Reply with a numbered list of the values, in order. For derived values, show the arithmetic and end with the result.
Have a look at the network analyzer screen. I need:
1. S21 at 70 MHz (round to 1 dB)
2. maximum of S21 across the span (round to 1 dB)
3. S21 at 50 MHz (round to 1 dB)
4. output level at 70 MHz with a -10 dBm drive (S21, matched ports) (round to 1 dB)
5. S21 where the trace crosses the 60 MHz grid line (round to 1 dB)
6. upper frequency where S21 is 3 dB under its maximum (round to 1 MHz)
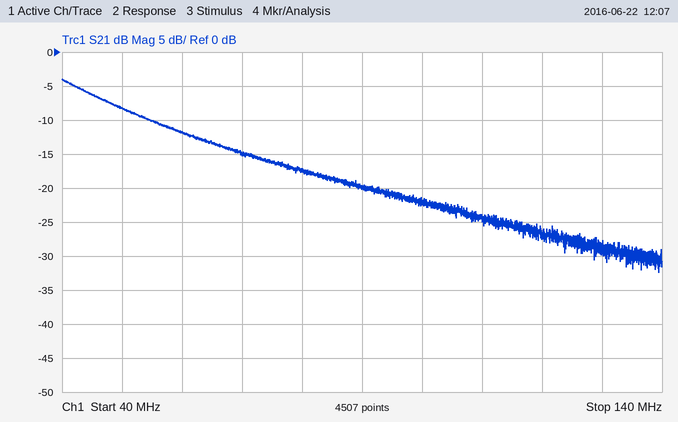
1. -15 dB
2. -4 dB
3. -8 dB
4. -10 dBm + (-15 dB) = -25 dBm
5. -12 dB
6. 47 MHz
